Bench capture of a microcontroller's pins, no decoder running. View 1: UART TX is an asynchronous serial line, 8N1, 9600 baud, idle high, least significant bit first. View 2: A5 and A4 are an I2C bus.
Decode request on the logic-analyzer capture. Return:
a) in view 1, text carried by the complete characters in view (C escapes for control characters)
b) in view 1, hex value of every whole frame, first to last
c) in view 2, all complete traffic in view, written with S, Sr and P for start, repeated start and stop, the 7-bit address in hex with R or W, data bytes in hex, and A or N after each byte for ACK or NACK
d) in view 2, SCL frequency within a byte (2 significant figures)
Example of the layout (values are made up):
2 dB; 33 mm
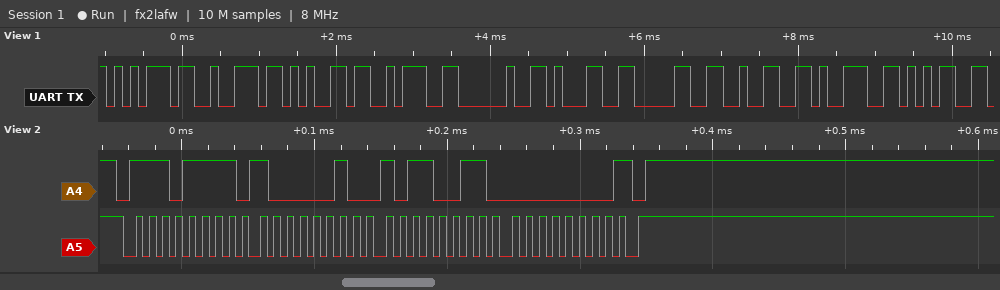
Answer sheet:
"ure: 10295"; 75 72 65 3A 20 31 30 32 39 35; S 77R A 82 A B3 A 00 N P; 100 kHz
